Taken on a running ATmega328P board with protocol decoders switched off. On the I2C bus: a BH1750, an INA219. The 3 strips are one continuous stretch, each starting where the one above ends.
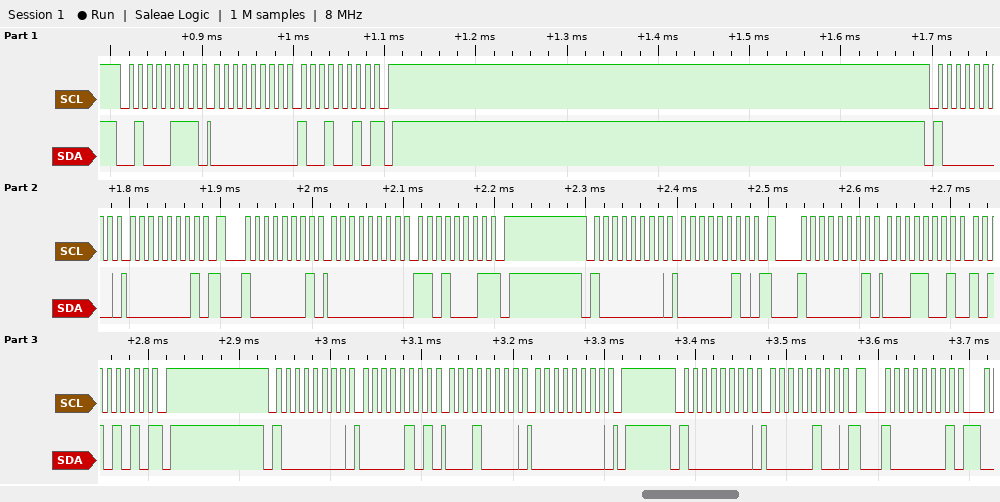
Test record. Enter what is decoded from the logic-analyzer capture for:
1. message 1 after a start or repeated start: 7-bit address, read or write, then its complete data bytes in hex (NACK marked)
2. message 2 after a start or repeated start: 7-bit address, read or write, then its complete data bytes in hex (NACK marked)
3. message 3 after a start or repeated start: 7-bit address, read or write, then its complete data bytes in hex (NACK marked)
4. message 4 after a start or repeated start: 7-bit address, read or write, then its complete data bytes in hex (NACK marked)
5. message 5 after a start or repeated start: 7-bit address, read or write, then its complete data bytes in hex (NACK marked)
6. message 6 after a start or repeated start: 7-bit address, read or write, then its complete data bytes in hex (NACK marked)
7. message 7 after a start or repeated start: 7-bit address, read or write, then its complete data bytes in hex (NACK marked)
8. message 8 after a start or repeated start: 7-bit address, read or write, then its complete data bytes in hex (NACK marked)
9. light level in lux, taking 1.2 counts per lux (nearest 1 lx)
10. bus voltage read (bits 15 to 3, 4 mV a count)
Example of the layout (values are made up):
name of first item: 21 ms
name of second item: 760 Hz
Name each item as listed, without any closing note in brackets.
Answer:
message 1 after a start or repeated start: 7-bit address, read or write, then its complete data bytes in hex: 0x23 read: 00 92 NACK
message 2 after a start or repeated start: 7-bit address, read or write, then its complete data bytes in hex: 0x40 write: 01
message 3 after a start or repeated start: 7-bit address, read or write, then its complete data bytes in hex: 0x40 read: 00 D1 NACK
message 4 after a start or repeated start: 7-bit address, read or write, then its complete data bytes in hex: 0x40 write: 02
message 5 after a start or repeated start: 7-bit address, read or write, then its complete data bytes in hex: 0x40 read: 19 AA NACK
message 6 after a start or repeated start: 7-bit address, read or write, then its complete data bytes in hex: 0x40 write: 05 10 00
message 7 after a start or repeated start: 7-bit address, read or write, then its complete data bytes in hex: 0x40 write: 04
message 8 after a start or repeated start: 7-bit address, read or write, then its complete data bytes in hex: 0x40 read
light level in lux, taking 1.2 counts per lux: 122 lx
bus voltage read: 3.284 V
